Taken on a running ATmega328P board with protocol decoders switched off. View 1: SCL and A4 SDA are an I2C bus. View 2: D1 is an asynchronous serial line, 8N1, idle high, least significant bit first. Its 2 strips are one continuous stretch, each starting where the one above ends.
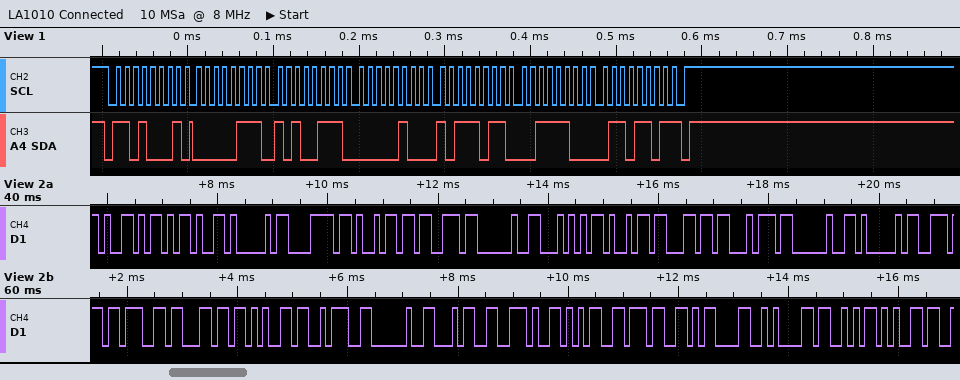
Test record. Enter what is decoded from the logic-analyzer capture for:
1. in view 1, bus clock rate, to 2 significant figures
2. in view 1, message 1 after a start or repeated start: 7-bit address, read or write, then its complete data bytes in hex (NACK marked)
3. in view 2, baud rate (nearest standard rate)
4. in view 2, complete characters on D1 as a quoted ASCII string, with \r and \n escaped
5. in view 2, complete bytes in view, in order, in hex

100 kHz
0x68 read: 07 A7 04 BB 3C 6D NACK
9600 baud
"Y-Axis Tilt Angle: 4.57\r\nSe"
59 2D 41 78 69 73 20 54 69 6C 74 20 41 6E 67 6C 65 3A 20 34 2E 35 37 0D 0A 53 65
